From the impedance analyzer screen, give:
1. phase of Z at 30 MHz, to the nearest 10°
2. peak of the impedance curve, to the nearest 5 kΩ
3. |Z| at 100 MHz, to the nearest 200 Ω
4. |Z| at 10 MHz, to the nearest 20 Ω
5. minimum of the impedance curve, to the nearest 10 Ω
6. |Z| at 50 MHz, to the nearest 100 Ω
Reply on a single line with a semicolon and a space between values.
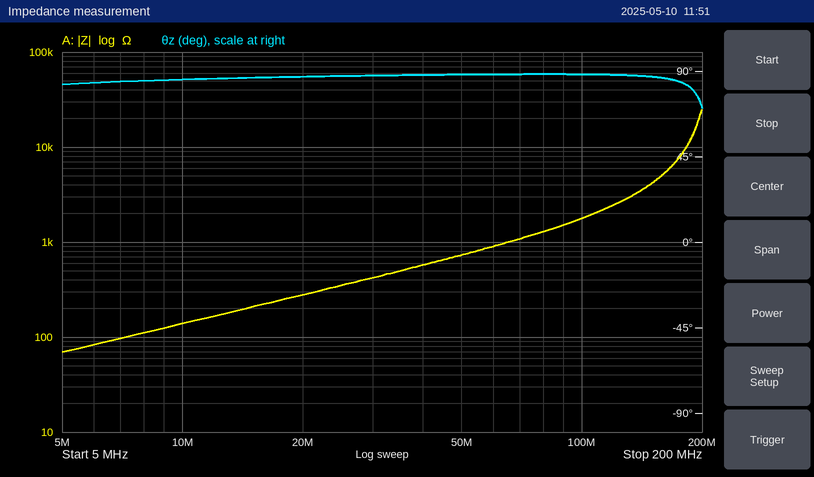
90°; 25 kΩ; 1.8 kΩ; 140 Ω; 70 Ω; 700 Ω
